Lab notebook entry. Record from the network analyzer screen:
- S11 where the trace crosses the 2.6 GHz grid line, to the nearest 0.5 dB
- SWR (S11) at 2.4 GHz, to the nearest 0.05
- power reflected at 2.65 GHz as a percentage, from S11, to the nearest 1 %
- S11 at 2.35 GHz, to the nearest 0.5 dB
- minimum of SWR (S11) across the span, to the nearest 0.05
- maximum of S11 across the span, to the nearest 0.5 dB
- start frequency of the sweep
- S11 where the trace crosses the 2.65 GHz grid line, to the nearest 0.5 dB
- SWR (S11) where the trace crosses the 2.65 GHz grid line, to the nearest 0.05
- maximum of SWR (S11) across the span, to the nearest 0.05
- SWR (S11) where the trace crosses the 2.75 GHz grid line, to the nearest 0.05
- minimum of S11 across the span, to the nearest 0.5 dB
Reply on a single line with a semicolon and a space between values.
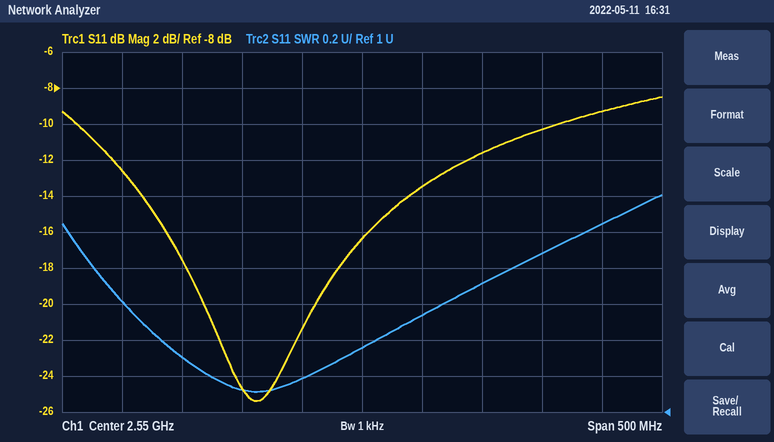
-13.5 dB; 1.30; 7 %; -12.5 dB; 1.10; -8.5 dB; 2.3 GHz; -11.5 dB; 1.70; 2.20; 2.05; -25.5 dB
